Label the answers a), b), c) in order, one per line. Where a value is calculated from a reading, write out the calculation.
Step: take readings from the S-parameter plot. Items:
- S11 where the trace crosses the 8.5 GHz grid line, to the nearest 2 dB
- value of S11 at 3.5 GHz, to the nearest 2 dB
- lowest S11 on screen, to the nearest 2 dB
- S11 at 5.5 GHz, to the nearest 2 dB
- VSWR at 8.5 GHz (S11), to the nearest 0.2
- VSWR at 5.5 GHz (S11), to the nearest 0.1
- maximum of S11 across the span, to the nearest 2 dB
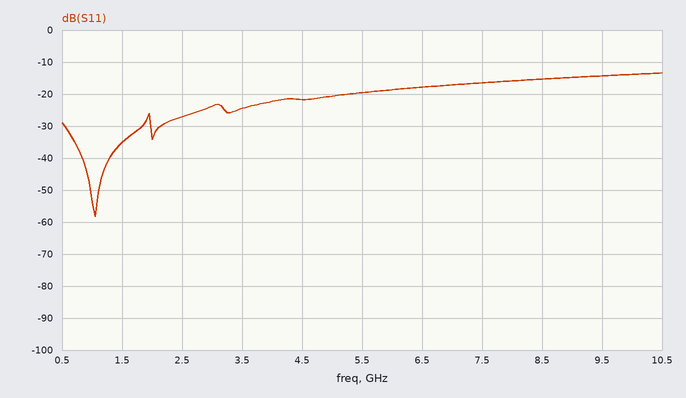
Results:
a) -16 dB
b) -24 dB
c) -58 dB
d) -20 dB
e) |Γ| = 10^(-16/20) = 0.1585; VSWR = (1 + 0.1585)/(1 − 0.1585) ≈ 1.4
f) |Γ| = 10^(-20/20) = 0.1000; VSWR = (1 + 0.1000)/(1 − 0.1000) ≈ 1.2
g) -14 dB
